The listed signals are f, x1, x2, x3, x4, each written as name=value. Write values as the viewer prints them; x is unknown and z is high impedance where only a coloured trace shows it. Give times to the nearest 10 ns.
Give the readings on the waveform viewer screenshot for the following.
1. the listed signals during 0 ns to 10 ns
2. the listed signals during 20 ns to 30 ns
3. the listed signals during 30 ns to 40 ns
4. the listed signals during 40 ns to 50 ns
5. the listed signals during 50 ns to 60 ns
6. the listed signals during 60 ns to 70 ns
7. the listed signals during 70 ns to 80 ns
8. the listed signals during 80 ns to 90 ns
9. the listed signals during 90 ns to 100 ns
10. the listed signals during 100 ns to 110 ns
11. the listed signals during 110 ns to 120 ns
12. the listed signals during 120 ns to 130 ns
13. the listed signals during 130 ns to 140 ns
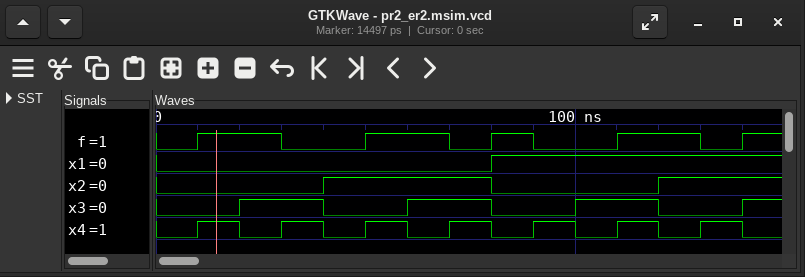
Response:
f=0, x1=0, x2=0, x3=0, x4=0
f=1, x1=0, x2=0, x3=1, x4=0
f=0, x1=0, x2=0, x3=1, x4=1
f=0, x1=0, x2=1, x3=0, x4=0
f=1, x1=0, x2=1, x3=0, x4=1
f=1, x1=0, x2=1, x3=1, x4=0
f=0, x1=0, x2=1, x3=1, x4=1
f=1, x1=1, x2=0, x3=0, x4=0
f=0, x1=1, x2=0, x3=0, x4=1
f=0, x1=1, x2=0, x3=1, x4=0
f=1, x1=1, x2=0, x3=1, x4=1
f=1, x1=1, x2=1, x3=0, x4=0
f=0, x1=1, x2=1, x3=0, x4=1
